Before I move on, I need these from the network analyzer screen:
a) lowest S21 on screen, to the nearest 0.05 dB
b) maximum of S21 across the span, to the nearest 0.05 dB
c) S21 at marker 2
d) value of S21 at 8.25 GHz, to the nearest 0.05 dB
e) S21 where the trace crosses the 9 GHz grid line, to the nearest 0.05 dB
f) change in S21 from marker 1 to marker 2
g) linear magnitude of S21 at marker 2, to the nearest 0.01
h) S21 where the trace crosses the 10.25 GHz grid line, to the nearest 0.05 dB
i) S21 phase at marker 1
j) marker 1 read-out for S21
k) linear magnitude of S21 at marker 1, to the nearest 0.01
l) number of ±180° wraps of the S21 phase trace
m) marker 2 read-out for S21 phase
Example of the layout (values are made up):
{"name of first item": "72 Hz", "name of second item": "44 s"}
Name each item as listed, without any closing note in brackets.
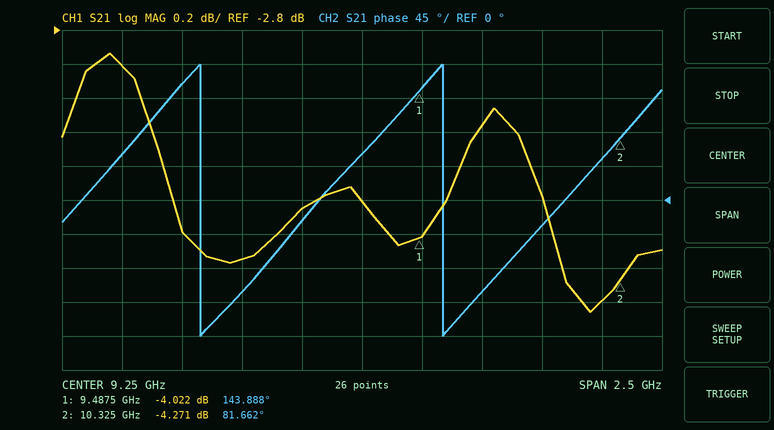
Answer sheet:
{"lowest S21 on screen, to the nearest 0.05 dB": "-4.45 dB", "maximum of S21 across the span, to the nearest 0.05 dB": "-2.95 dB", "S21 at marker 2": "-4.271 dB", "value of S21 at 8.25 GHz, to the nearest 0.05 dB": "-3.00 dB", "S21 where the trace crosses the 9 GHz grid line, to the nearest 0.05 dB": "-3.85 dB", "change in S21 from marker 1 to marker 2": "-0.249 dB", "linear magnitude of S21 at marker 2, to the nearest 0.01": "0.61", "S21 where the trace crosses the 10.25 GHz grid line, to the nearest 0.05 dB": "-4.40 dB", "S21 phase at marker 1": "143.888°", "marker 1 read-out for S21": "-4.022 dB", "linear magnitude of S21 at marker 1, to the nearest 0.01": "0.63", "number of ±180° wraps of the S21 phase trace": "2", "marker 2 read-out for S21 phase": "81.662°"}
